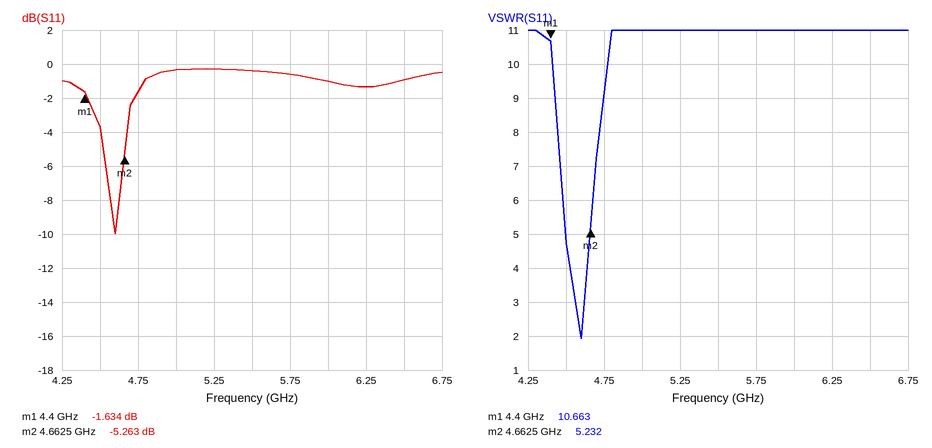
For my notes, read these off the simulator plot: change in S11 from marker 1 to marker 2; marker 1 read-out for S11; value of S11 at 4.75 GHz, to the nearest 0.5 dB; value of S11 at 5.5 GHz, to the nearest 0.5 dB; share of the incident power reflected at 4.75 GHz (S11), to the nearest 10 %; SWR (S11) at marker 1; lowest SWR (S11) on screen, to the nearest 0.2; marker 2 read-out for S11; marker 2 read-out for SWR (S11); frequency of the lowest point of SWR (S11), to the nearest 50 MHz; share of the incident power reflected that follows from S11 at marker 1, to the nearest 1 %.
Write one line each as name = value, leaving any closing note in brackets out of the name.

change in S11 from marker 1 to marker 2 = -3.629 dB
marker 1 read-out for S11 = -1.634 dB
value of S11 at 4.75 GHz, to the nearest 0.5 dB = -1.5 dB
value of S11 at 5.5 GHz, to the nearest 0.5 dB = -0.5 dB
share of the incident power reflected at 4.75 GHz (S11), to the nearest 10 % = 70 %
SWR (S11) at marker 1 = 10.663
lowest SWR (S11) on screen, to the nearest 0.2 = 2.0
marker 2 read-out for S11 = -5.263 dB
marker 2 read-out for SWR = 5.232
frequency of the lowest point of SWR (S11), to the nearest 50 MHz = 4.60 GHz
share of the incident power reflected that follows from S11 at marker 1, to the nearest 1 % = 69 %
